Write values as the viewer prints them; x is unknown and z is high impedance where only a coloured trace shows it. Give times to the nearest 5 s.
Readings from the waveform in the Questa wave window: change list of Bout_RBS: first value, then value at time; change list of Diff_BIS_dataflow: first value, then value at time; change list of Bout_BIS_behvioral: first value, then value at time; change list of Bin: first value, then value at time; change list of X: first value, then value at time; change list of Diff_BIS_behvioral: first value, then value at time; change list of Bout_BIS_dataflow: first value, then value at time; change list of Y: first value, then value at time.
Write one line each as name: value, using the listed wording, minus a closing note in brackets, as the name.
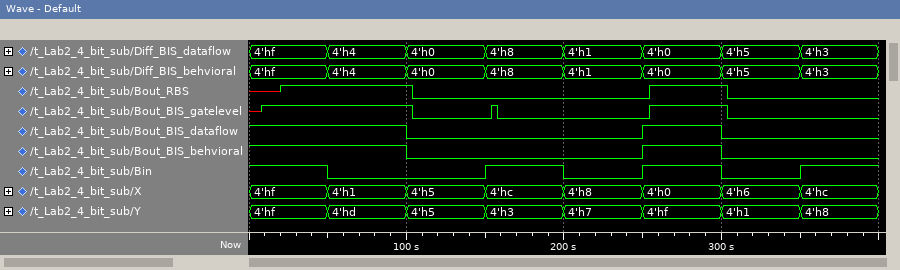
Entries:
change list of Bout_RBS: first value, then value at time: x, 1 at 20 s, 0 at 105 s, 1 at 255 s, 0 at 305 s
change list of Diff_BIS_dataflow: first value, then value at time: 4'hf, 4'h4 at 50 s, 4'h0 at 100 s, 4'h8 at 150 s, 4'h1 at 200 s, 4'h0 at 250 s, 4'h5 at 300 s, 4'h3 at 350 s
change list of Bout_BIS_behvioral: first value, then value at time: 1, 0 at 100 s, 1 at 250 s, 0 at 300 s
change list of Bin: first value, then value at time: 1, 0 at 50 s, 1 at 150 s, 0 at 200 s, 1 at 250 s, 0 at 300 s, 1 at 350 s
change list of X: first value, then value at time: 4'hf, 4'h1 at 50 s, 4'h5 at 100 s, 4'hc at 150 s, 4'h8 at 200 s, 4'h0 at 250 s, 4'h6 at 300 s, 4'hc at 350 s
change list of Diff_BIS_behvioral: first value, then value at time: 4'hf, 4'h4 at 50 s, 4'h0 at 100 s, 4'h8 at 150 s, 4'h1 at 200 s, 4'h0 at 250 s, 4'h5 at 300 s, 4'h3 at 350 s
change list of Bout_BIS_dataflow: first value, then value at time: 1, 0 at 100 s, 1 at 250 s, 0 at 300 s
change list of Y: first value, then value at time: 4'hf, 4'hd at 50 s, 4'h5 at 100 s, 4'h3 at 150 s, 4'h7 at 200 s, 4'hf at 250 s, 4'h1 at 300 s, 4'h8 at 350 s
